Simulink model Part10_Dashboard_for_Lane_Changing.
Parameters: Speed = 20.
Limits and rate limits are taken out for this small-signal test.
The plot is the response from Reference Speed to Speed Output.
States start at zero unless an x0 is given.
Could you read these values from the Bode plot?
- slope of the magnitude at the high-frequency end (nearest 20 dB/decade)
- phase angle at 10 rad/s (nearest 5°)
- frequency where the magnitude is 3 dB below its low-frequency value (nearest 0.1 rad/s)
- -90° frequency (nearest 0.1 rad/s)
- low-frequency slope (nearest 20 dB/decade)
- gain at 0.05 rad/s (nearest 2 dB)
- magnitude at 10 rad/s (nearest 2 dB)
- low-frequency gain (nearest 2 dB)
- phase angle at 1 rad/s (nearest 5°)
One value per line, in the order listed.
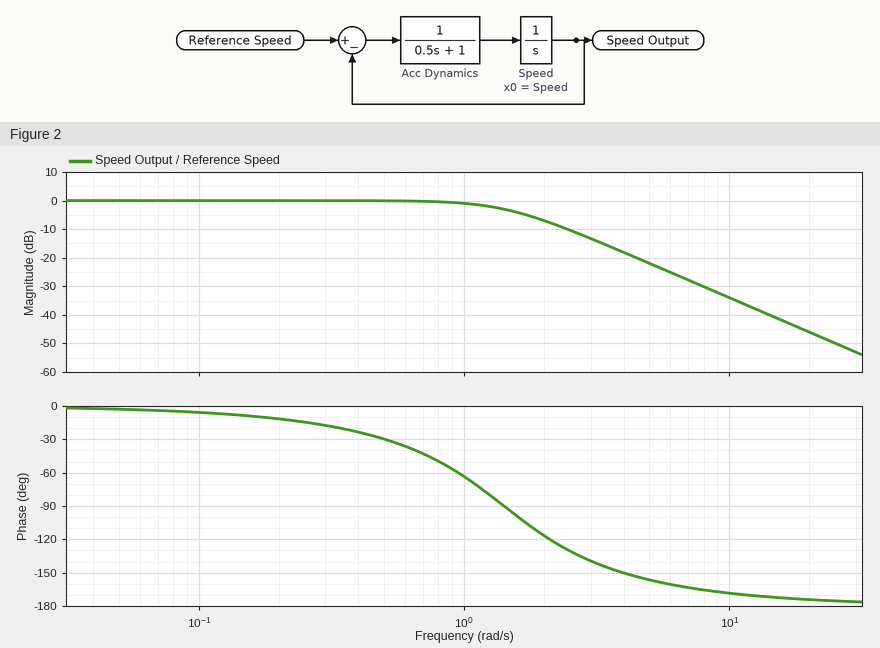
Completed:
-40 dB/decade
-170°
1.4 rad/s
1.4 rad/s
0 dB/decade
0 dB
-34 dB
0 dB
-65°
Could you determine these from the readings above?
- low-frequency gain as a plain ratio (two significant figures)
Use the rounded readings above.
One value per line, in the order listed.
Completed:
1.0
